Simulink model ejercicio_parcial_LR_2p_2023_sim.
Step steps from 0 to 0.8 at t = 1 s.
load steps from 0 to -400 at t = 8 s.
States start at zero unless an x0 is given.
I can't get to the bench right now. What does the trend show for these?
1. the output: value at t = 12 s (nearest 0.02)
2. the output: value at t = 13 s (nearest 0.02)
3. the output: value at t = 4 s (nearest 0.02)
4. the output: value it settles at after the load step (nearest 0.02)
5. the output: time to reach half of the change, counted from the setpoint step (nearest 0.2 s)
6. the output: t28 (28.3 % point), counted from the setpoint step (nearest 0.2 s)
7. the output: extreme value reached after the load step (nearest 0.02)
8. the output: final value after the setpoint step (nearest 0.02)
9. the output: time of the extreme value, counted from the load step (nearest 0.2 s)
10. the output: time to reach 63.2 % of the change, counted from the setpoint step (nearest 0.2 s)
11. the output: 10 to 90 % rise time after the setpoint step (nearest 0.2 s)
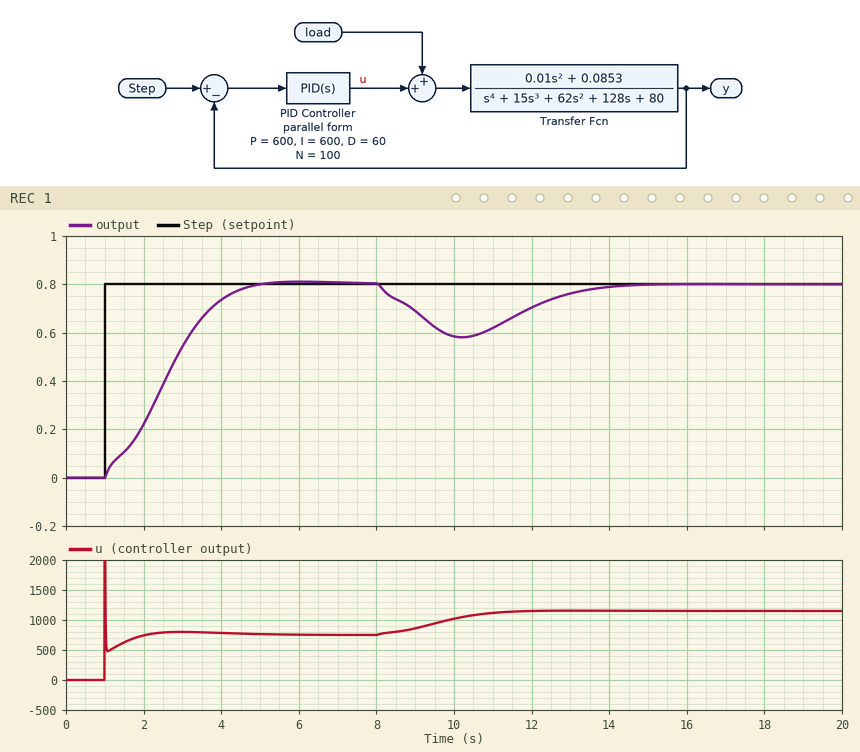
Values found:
0.70
0.76
0.74
0.80
1.6 s
1.0 s
0.58
0.80
2.2 s
1.8 s
2.6 s
